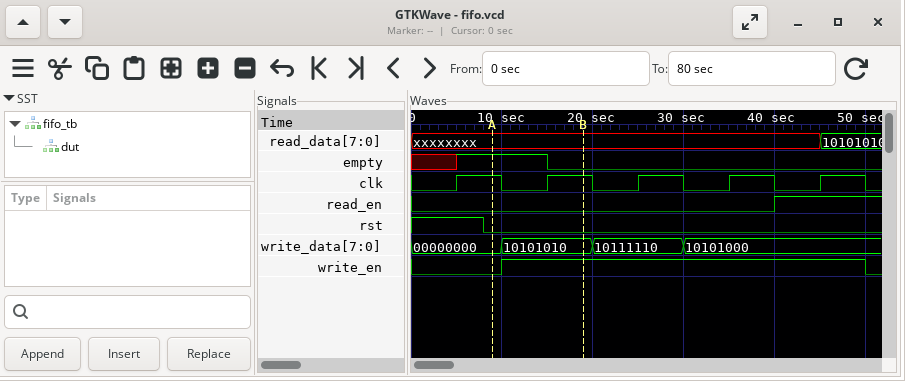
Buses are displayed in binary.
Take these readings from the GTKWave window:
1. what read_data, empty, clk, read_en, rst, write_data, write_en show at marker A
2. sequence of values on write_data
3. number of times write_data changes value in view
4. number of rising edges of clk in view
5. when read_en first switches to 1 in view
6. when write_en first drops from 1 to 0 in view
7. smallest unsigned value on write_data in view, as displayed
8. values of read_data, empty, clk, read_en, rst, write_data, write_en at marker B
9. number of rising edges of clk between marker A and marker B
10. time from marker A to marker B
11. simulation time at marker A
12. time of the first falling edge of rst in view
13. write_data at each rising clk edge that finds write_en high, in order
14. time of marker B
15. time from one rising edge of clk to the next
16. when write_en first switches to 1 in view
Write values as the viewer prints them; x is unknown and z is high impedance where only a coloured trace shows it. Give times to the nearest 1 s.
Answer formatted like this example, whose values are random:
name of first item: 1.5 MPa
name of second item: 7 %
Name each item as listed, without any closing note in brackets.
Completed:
what read_data, empty, clk, read_en, rst, write_data, write_en show at marker A: read_data=xxxxxxxx, empty=1, clk=1, read_en=0, rst=0, write_data=00000000, write_en=0
sequence of values on write_data: 00000000, 10101010, 10111110, 10101000
number of times write_data changes value in view: 3
number of rising edges of clk in view: 5
when read_en first switches to 1 in view: 40 s
when write_en first drops from 1 to 0 in view: 50 s
smallest unsigned value on write_data in view, as displayed: 00000000
values of read_data, empty, clk, read_en, rst, write_data, write_en at marker B: read_data=xxxxxxxx, empty=0, clk=1, read_en=0, rst=0, write_data=10101010, write_en=1
number of rising edges of clk between marker A and marker B: 1
time from marker A to marker B: 10 s
simulation time at marker A: 9 s
time of the first falling edge of rst in view: 8 s
write_data at each rising clk edge that finds write_en high, in order: 10101010, 10111110, 10101000, 10101000
time of marker B: 19 s
time from one rising edge of clk to the next: 10 s
when write_en first switches to 1 in view: 10 s
